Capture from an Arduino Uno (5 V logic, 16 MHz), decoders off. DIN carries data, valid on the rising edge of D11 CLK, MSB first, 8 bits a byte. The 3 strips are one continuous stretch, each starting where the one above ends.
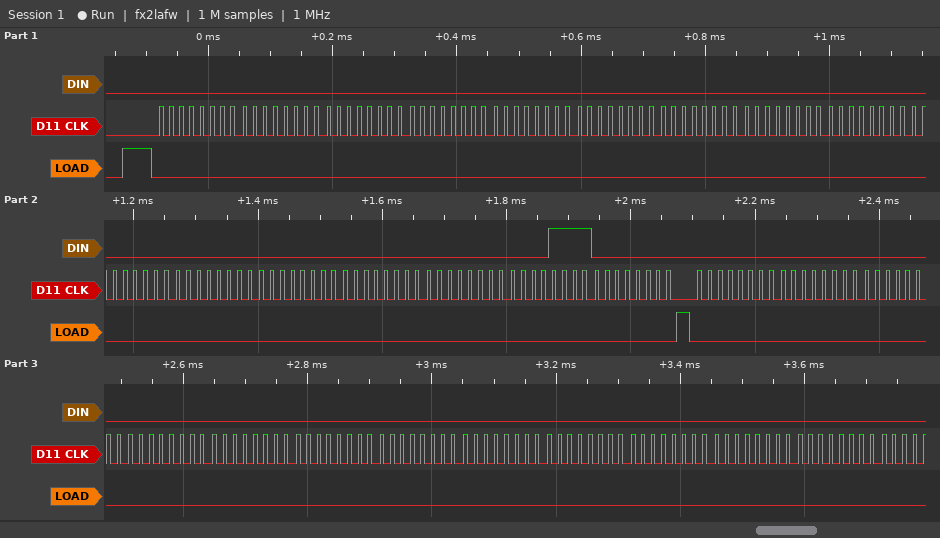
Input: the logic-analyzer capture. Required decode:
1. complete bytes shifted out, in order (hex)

00 00 00 00 00 00 00 00 00 00 00 00 00 00 0F 00 00 00 00 00 00 00 00 00 00 00 00 00
